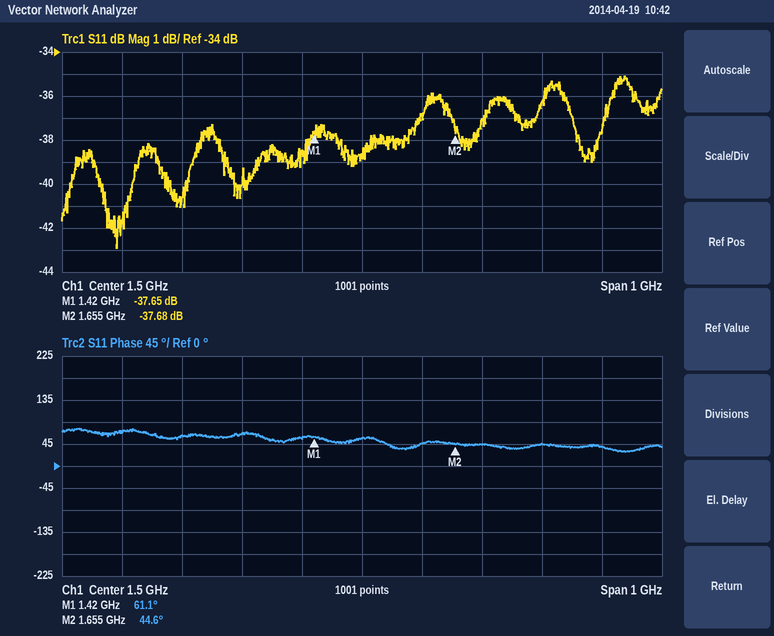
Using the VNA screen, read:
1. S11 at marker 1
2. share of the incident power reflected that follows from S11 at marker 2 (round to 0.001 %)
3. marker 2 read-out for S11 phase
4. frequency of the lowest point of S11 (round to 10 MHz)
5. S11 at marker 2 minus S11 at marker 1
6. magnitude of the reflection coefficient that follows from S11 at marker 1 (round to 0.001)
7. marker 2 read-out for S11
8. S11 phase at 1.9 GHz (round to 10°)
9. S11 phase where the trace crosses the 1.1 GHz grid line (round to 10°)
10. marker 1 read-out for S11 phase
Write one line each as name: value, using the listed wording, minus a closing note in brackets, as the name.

S11 at marker 1: -37.65 dB
share of the incident power reflected that follows from S11 at marker 2: 0.017 %
marker 2 read-out for S11 phase: 44.6°
frequency of the lowest point of S11: 1.09 GHz
S11 at marker 2 minus S11 at marker 1: -0.03 dB
magnitude of the reflection coefficient that follows from S11 at marker 1: 0.013
marker 2 read-out for S11: -37.68 dB
S11 phase at 1.9 GHz: 40°
S11 phase where the trace crosses the 1.1 GHz grid line: 70°
marker 1 read-out for S11 phase: 61.1°
